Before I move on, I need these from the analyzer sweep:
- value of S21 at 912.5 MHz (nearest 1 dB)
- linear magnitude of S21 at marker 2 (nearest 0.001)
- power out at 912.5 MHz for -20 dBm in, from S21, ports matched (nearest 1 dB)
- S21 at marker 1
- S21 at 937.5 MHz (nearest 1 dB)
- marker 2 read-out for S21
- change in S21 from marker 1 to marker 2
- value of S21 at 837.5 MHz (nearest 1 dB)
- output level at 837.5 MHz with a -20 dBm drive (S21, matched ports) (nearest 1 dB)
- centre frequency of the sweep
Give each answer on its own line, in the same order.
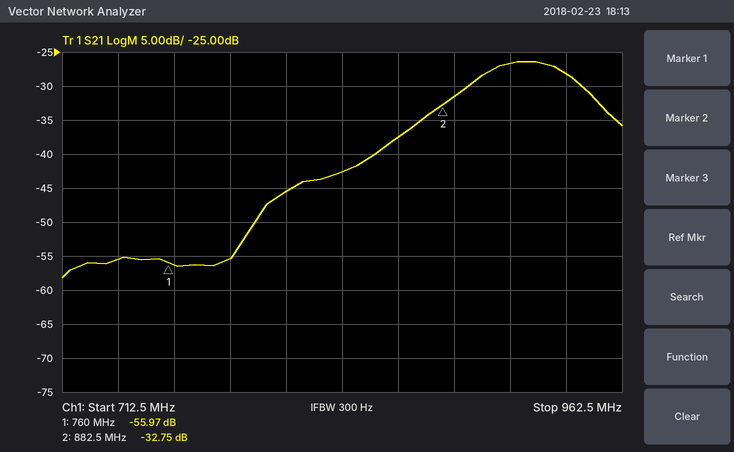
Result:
-27 dB
0.023
-47 dBm
-55.97 dB
-28 dB
-32.75 dB
23.22 dB
-43 dB
-63 dBm
837.5 MHz
